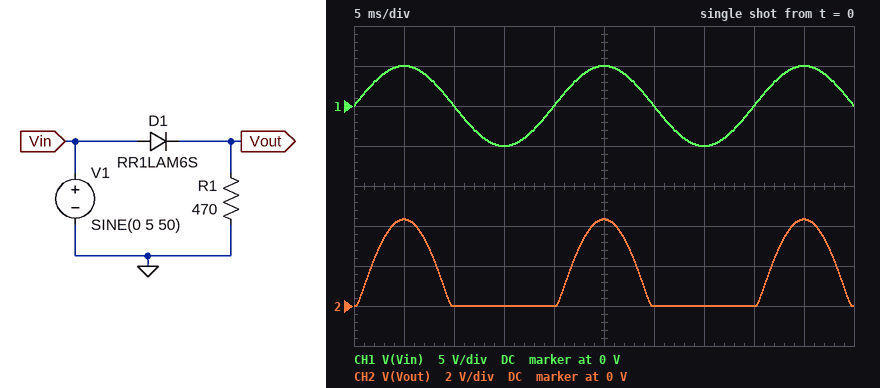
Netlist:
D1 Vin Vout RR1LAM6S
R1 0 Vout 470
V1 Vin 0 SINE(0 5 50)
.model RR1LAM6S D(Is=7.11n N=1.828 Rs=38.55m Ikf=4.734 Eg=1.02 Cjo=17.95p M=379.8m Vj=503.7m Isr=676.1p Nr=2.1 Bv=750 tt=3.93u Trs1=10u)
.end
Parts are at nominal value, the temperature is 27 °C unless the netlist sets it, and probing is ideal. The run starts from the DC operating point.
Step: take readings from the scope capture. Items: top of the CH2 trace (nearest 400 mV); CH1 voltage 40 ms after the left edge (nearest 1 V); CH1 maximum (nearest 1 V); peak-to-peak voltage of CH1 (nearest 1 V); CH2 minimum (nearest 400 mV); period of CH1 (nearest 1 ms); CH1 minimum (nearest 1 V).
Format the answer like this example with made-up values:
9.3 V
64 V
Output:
4.4 V
0 V
5 V
10 V
0 V
20 ms
-5 V
